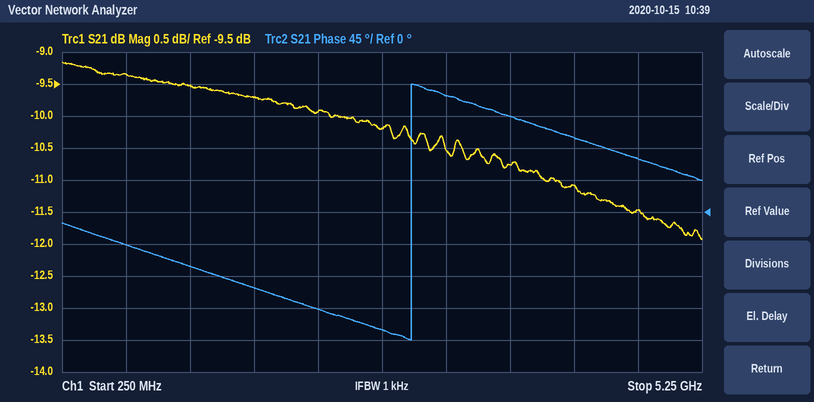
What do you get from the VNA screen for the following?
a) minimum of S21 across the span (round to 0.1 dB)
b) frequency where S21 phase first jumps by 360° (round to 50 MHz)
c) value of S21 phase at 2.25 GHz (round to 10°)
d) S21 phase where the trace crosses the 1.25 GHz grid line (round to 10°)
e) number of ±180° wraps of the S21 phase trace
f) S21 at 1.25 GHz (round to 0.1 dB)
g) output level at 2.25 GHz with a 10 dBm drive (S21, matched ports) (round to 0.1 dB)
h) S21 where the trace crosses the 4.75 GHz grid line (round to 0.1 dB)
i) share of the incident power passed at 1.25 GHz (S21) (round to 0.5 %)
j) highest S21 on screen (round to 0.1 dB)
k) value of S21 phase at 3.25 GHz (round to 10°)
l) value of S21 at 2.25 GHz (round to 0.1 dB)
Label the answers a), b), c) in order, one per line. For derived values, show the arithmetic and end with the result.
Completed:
a) -11.9 dB
b) 3.00 GHz
c) -140°
d) -80°
e) 1
f) -9.5 dB
g) 10 dBm + (-9.9 dB) = 0.1 dBm
h) -11.5 dB
i) 10^(-9.5/10) ≈ 11.2 %, so 11.0 % to the nearest 0.5 %
j) -9.2 dB
k) 160°
l) -9.9 dB
